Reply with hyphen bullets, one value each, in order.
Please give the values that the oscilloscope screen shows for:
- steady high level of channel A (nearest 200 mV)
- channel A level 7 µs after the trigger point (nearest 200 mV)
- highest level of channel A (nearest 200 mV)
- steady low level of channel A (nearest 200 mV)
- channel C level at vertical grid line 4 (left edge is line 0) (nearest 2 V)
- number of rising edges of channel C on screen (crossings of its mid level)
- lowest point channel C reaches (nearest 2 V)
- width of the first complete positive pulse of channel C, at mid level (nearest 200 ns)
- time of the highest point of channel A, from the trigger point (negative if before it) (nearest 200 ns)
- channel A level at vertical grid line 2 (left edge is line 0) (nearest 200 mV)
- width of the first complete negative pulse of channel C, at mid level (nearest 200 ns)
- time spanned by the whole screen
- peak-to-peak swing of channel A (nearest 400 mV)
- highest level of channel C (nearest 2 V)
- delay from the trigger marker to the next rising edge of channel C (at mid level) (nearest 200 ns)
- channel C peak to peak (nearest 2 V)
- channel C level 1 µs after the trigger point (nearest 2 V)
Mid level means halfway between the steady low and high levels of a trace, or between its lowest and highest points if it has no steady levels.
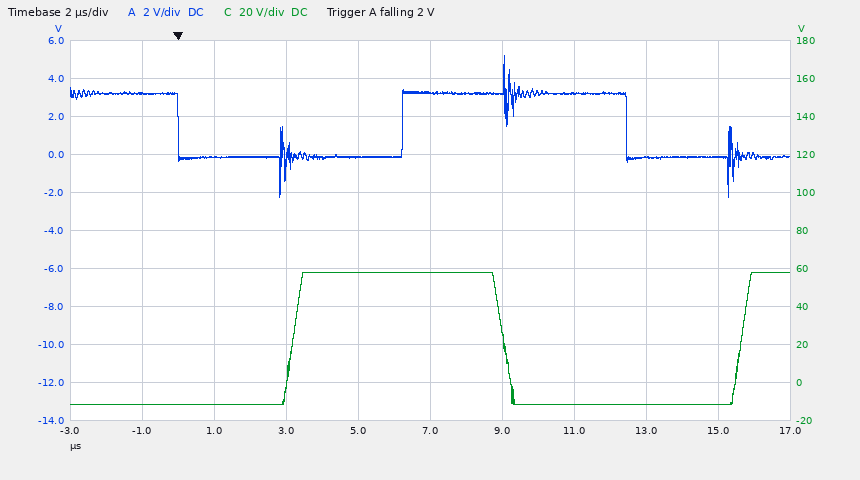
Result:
- 3.2 V
- 3.2 V
- 5.2 V
- -200 mV
- 58 V
- 2
- -12 V
- 5.8 µs
- +9.0 µs
- -200 mV
- 6.6 µs
- 20 µs
- 7.6 V
- 58 V
- 3.2 µs
- 70 V
- -12 V
